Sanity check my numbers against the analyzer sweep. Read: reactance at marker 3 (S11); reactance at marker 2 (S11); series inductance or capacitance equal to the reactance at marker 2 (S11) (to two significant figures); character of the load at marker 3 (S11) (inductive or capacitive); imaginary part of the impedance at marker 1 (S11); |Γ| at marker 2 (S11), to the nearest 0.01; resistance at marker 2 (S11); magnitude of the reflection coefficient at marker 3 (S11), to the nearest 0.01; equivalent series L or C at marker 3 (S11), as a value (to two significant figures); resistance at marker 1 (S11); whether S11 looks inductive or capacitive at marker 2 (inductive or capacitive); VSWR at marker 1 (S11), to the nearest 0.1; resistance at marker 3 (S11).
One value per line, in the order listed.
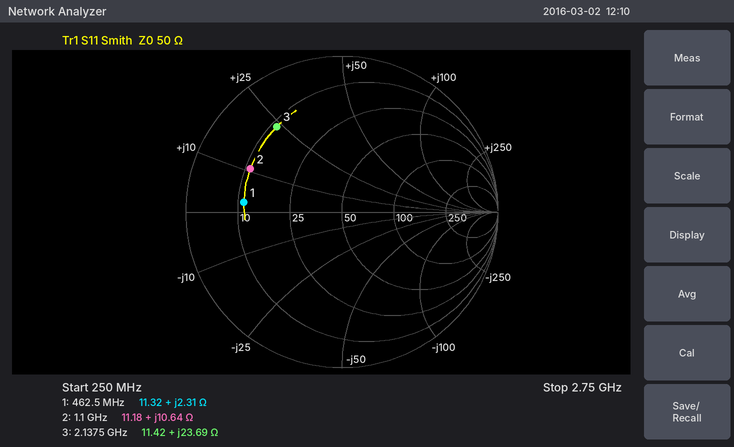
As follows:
+23.69 Ω
+10.64 Ω
1.5 nH
inductive
+2.31 Ω
0.65
11.18 Ω
0.69
1.8 nH
11.32 Ω
inductive
4.4
11.42 Ω
